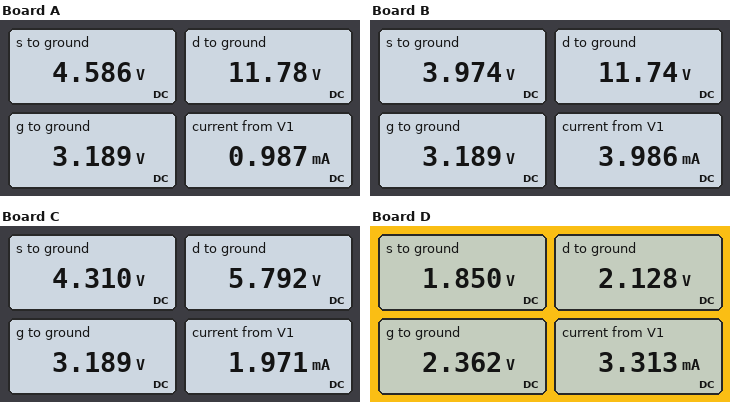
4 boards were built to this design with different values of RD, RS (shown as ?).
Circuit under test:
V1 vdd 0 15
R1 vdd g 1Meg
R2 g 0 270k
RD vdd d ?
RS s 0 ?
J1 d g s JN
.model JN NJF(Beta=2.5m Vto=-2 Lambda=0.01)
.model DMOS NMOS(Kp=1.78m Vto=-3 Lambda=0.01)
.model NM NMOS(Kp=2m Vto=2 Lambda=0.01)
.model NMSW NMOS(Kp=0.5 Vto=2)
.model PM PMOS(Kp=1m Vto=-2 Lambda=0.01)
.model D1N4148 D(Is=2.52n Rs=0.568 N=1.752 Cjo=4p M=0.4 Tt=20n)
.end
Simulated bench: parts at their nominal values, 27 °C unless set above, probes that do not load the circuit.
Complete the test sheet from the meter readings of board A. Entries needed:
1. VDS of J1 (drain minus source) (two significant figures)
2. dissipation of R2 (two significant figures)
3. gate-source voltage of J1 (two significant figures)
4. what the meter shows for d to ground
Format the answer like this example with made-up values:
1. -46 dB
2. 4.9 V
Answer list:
1. 7.2 V
2. 38 µW
3. -1.4 V
4. 11.78 V
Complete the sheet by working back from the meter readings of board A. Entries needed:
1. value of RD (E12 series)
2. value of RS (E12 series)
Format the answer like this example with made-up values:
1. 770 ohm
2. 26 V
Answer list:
1. 3.3 kΩ
2. 4.7 kΩ
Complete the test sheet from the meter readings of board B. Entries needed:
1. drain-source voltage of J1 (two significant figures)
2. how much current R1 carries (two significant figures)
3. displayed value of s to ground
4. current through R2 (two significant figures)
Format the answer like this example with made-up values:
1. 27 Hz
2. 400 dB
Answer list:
1. 7.8 V
2. 12 µA
3. 3.974 V
4. 12 µA
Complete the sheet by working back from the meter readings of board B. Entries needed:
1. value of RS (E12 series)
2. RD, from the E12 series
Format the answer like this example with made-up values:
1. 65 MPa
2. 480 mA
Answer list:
1. 1 kΩ
2. 820 Ω
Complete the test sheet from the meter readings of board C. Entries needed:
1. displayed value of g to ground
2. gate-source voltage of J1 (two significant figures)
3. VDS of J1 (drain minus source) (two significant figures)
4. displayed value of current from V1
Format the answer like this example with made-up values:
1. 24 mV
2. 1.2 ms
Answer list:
1. 3.189 V
2. -1.1 V
3. 1.5 V
4. 1.971 mA
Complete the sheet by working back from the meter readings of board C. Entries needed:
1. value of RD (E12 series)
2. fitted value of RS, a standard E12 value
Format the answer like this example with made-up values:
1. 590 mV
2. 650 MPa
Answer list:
1. 4.7 kΩ
2. 2.2 kΩ
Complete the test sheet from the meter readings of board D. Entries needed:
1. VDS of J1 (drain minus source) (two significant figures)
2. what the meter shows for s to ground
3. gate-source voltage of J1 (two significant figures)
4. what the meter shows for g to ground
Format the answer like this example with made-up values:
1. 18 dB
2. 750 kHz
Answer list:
1. 280 mV
2. 1.850 V
3. 510 mV
4. 2.362 V
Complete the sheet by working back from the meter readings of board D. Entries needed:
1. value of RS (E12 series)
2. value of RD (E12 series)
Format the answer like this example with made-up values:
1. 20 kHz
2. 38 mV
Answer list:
1. 560 Ω
2. 3.9 kΩ
